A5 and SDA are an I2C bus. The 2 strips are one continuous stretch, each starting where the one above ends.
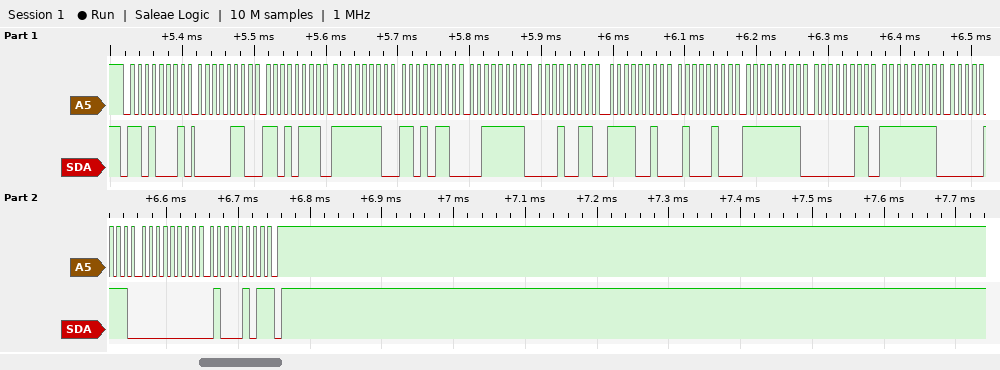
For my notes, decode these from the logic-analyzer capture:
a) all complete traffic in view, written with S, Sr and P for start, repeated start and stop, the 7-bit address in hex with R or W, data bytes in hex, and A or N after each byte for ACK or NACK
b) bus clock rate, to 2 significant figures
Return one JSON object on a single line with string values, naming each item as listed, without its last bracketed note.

{"all complete traffic in view, written with S, Sr and P for start, repeated start and stop, the 7-bit address in hex with R or W, data bytes in hex, and A or N after each byte for ACK or NACK": "S 68R A 06 A D7 A FE A D6 A 3F A 13 A F2 A 44 A FF A 03 A FF A 07 A 00 A 45 N P", "bus clock rate, to 2 significant figures": "100 kHz"}
